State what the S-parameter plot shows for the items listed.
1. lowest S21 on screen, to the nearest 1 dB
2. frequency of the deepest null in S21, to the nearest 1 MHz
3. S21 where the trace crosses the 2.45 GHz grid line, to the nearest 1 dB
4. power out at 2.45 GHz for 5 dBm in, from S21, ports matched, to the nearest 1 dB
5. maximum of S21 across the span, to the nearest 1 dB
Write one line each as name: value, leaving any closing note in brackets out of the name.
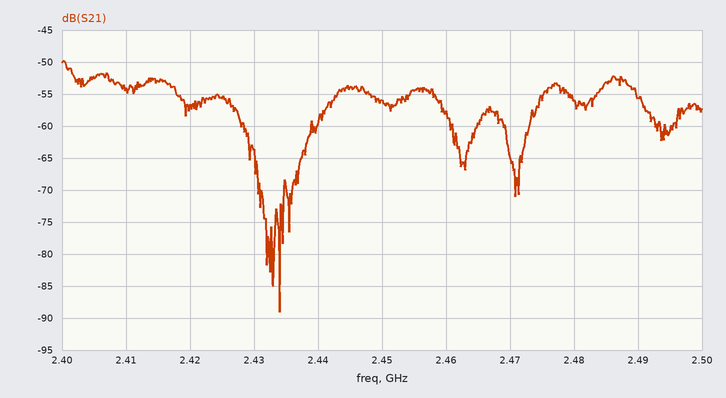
lowest S21 on screen, to the nearest 1 dB: -89 dB
frequency of the deepest null in S21, to the nearest 1 MHz: 2.434 GHz
S21 where the trace crosses the 2.45 GHz grid line, to the nearest 1 dB: -56 dB
power out at 2.45 GHz for 5 dBm in, from S21, ports matched, to the nearest 1 dB: -51 dBm
maximum of S21 across the span, to the nearest 1 dB: -50 dB
